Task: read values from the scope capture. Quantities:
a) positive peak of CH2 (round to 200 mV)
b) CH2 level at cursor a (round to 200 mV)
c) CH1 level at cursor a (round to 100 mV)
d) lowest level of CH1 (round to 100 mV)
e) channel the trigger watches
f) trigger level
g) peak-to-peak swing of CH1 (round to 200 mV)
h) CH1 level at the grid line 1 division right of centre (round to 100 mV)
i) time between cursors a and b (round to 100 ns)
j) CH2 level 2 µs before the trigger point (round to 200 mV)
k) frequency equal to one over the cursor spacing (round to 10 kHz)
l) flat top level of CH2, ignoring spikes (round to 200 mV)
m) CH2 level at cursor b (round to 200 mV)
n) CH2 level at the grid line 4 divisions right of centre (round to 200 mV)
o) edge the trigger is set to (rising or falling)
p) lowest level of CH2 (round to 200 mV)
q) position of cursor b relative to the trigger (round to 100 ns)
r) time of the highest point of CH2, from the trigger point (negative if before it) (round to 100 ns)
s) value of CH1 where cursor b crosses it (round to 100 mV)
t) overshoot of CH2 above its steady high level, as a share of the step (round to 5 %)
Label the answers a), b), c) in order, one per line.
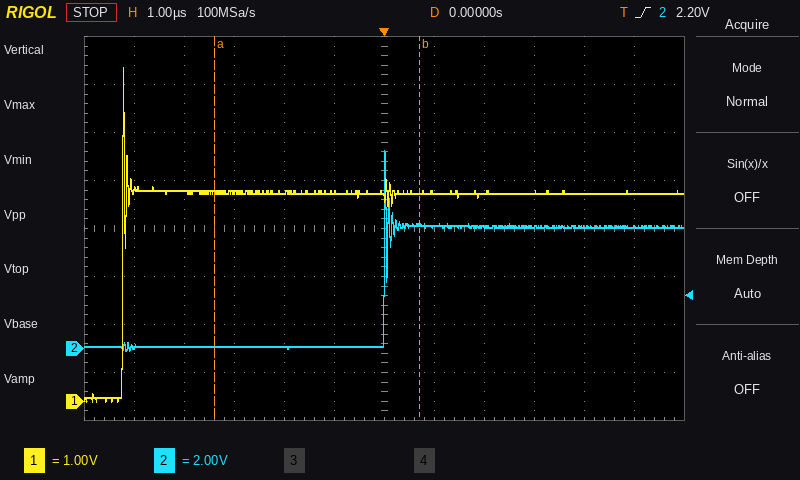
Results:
a) 8.2 V
b) 0.0 V
c) 4.4 V
d) 0.0 V
e) CH2
f) 2.20 V
g) 7.0 V
h) 4.4 V
i) 4.1 µs
j) 0.0 V
k) 240 kHz
l) 5.0 V
m) 5.2 V
n) 5.0 V
o) rising
p) 0.0 V
q) +700 ns
r) 0.0 µs
s) 4.4 V
t) 65 %
